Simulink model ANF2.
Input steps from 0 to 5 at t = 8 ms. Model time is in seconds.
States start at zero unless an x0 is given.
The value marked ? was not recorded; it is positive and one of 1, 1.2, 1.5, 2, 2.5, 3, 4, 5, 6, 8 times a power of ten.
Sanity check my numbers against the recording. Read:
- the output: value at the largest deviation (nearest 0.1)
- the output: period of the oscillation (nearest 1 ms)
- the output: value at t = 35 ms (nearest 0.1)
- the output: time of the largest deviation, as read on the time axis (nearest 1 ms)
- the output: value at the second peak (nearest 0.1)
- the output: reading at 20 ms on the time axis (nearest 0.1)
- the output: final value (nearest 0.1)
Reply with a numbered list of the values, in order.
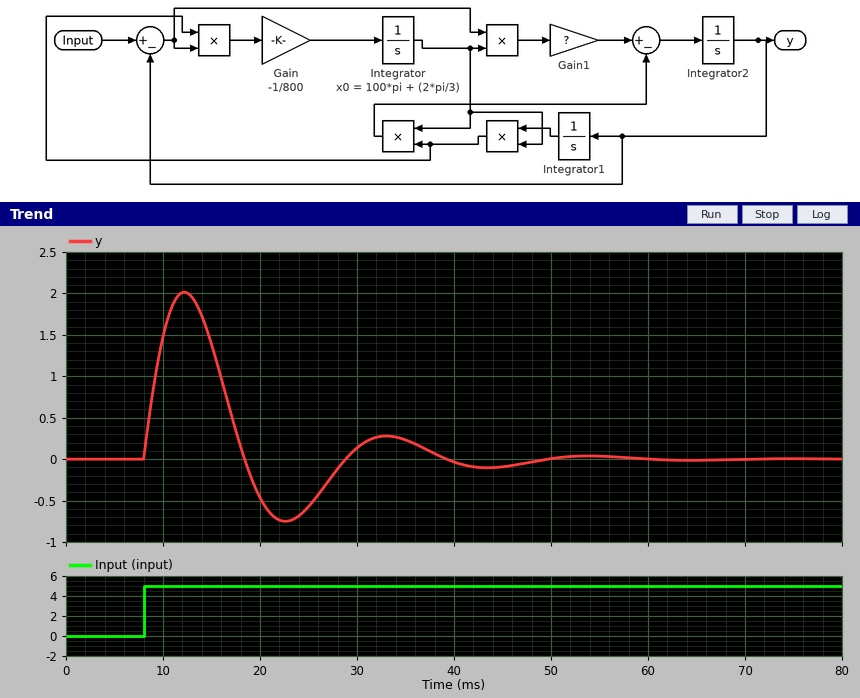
1. 2.0
2. 21 ms
3. 0.2
4. 12 ms
5. 0.3
6. -0.5
7. 0.0
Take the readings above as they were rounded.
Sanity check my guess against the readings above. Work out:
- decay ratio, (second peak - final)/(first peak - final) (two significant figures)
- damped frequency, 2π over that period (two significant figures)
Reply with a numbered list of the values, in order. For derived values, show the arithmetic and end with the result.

1. (0.3 - 0) / (2 - 0) = 0.15
2. 2π / 21 = 0.30 rad/ms
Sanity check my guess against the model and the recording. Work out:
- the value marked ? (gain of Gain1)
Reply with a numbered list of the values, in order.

1. 0.6
